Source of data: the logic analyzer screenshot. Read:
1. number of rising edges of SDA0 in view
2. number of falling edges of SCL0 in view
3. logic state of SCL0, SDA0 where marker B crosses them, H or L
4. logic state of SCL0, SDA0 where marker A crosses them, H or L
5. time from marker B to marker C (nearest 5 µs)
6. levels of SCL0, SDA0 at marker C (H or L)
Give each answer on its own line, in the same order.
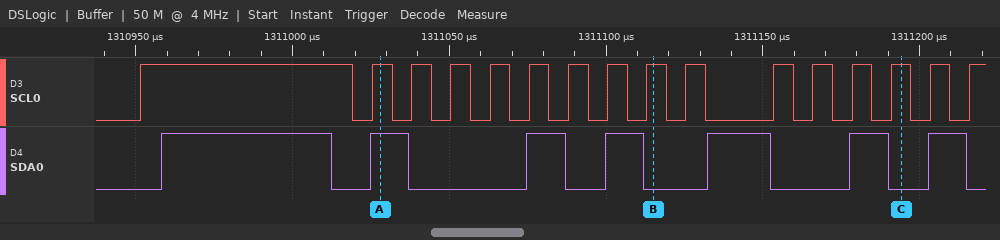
7
15
SCL0=H, SDA0=L
SCL0=H, SDA0=H
80 µs
SCL0=H, SDA0=L
